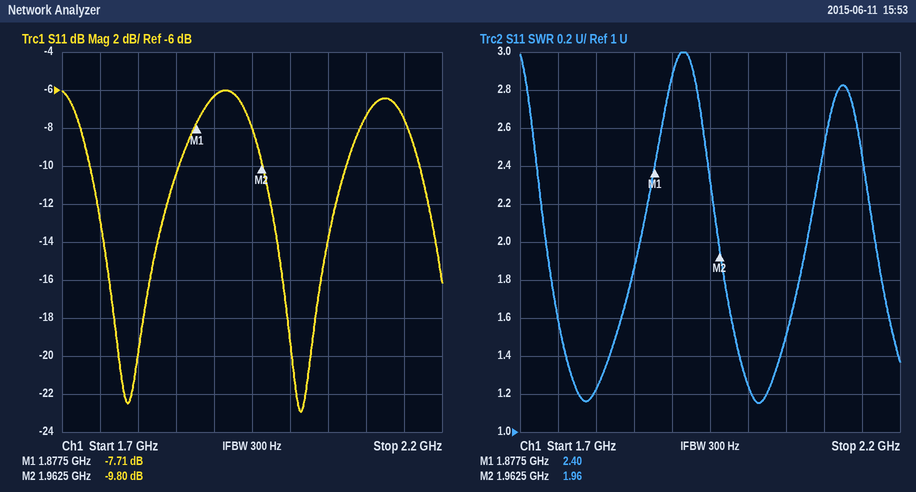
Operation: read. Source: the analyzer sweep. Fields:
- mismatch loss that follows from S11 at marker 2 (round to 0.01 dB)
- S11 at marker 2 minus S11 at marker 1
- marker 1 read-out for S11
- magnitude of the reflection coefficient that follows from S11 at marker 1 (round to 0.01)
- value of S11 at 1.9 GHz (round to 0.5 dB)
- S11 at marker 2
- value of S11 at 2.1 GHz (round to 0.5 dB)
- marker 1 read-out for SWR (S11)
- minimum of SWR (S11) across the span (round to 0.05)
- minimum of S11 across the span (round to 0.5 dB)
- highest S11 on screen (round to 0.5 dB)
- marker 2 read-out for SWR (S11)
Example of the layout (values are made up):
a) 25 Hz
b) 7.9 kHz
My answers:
a) 0.48 dB
b) -2.09 dB
c) -7.71 dB
d) 0.41
e) -6.5 dB
f) -9.80 dB
g) -7.5 dB
h) 2.40
i) 1.15
j) -23.0 dB
k) -6.0 dB
l) 1.96
